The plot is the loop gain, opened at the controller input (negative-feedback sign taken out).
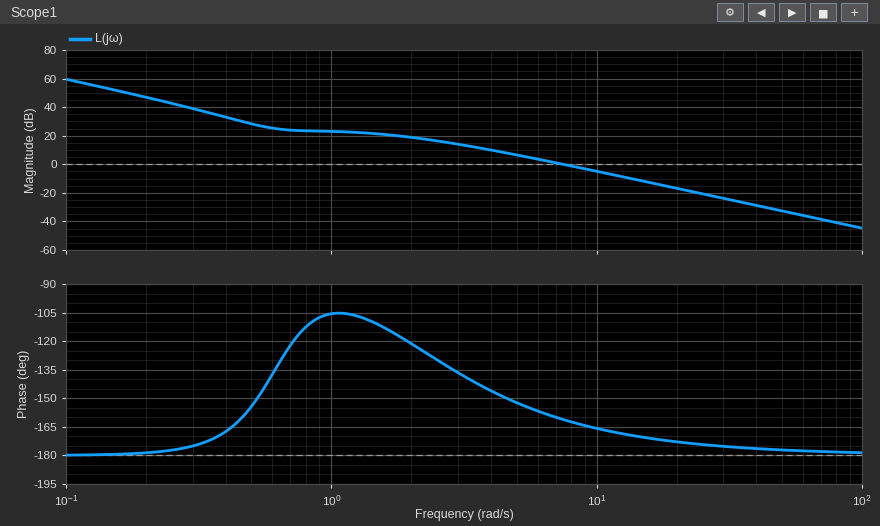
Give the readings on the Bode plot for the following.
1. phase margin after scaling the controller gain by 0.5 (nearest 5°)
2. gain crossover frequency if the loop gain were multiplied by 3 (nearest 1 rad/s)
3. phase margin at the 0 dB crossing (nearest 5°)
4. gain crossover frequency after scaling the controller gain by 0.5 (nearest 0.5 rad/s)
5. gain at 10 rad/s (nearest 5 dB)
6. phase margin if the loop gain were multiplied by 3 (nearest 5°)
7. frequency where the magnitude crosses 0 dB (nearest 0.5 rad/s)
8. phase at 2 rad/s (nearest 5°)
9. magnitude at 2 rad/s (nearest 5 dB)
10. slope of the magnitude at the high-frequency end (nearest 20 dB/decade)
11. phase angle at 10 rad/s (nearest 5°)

25°
13 rad/s
20°
5.0 rad/s
-5 dB
10°
7.5 rad/s
-120°
20 dB
-40 dB/decade
-165°
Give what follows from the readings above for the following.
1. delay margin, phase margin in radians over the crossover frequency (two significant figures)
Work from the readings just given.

0.047 s
